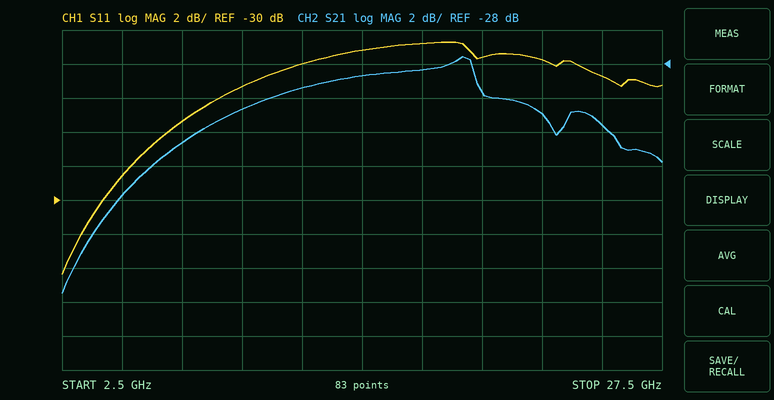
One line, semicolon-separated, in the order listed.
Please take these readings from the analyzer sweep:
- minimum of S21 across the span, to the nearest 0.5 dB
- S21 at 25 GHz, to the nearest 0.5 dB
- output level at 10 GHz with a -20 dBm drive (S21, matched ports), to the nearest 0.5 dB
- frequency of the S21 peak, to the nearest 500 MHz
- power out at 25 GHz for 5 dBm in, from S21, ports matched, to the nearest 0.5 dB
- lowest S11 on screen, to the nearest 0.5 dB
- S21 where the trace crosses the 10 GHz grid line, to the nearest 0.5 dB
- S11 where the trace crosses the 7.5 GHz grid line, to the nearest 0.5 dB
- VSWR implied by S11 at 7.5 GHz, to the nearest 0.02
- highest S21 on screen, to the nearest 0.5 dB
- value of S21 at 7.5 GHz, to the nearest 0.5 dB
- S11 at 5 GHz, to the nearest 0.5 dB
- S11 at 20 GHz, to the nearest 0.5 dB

-41.5 dB; -31.5 dB; -50.5 dBm; 19.0 GHz; -26.5 dBm; -34.5 dB; -30.5 dB; -25.5 dB; 1.12; -27.5 dB; -32.5 dB; -28.5 dB; -21.5 dB
